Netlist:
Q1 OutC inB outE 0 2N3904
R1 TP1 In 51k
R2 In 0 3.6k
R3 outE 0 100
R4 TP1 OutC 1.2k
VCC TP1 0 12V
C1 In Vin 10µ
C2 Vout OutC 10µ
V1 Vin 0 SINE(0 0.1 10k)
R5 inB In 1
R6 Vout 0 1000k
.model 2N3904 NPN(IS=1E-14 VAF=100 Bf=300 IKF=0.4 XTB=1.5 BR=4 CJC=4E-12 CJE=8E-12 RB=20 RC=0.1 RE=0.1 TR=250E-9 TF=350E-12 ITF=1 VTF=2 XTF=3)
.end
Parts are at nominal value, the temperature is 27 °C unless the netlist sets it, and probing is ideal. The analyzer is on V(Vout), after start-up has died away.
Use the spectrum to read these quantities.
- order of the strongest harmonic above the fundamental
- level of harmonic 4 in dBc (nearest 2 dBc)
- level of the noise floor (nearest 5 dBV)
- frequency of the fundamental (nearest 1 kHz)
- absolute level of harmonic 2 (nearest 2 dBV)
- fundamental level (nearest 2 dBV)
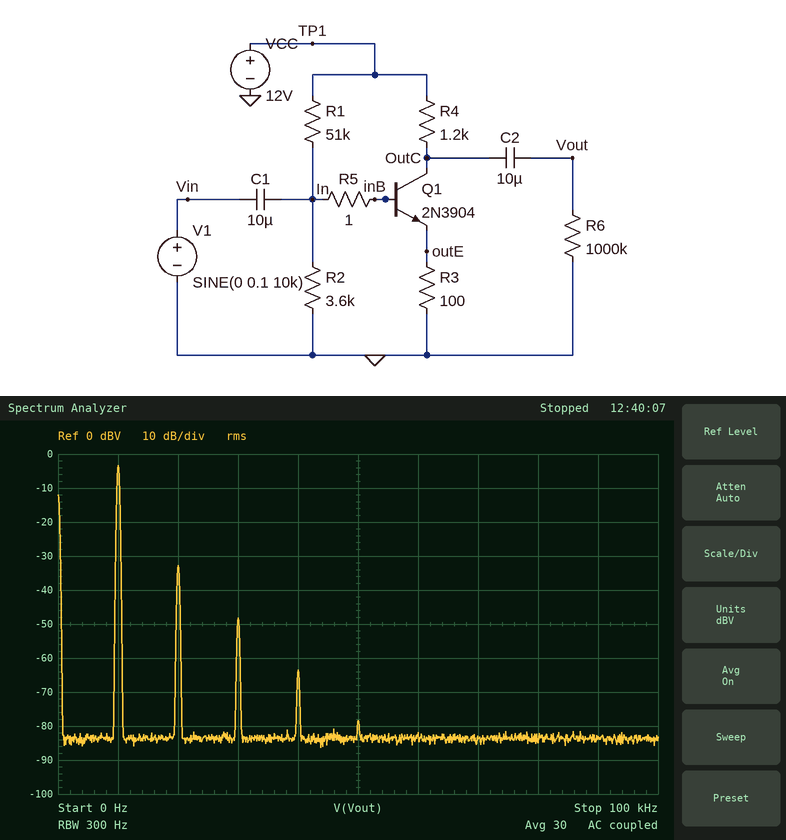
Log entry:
2
-60 dBc
-85 dBV
10 kHz
-32 dBV
-4 dBV
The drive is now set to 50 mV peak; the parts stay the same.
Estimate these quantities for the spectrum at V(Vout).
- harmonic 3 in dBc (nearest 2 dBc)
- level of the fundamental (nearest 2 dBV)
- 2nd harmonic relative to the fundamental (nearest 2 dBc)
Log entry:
-58 dBc
-10 dBV
-36 dBc
